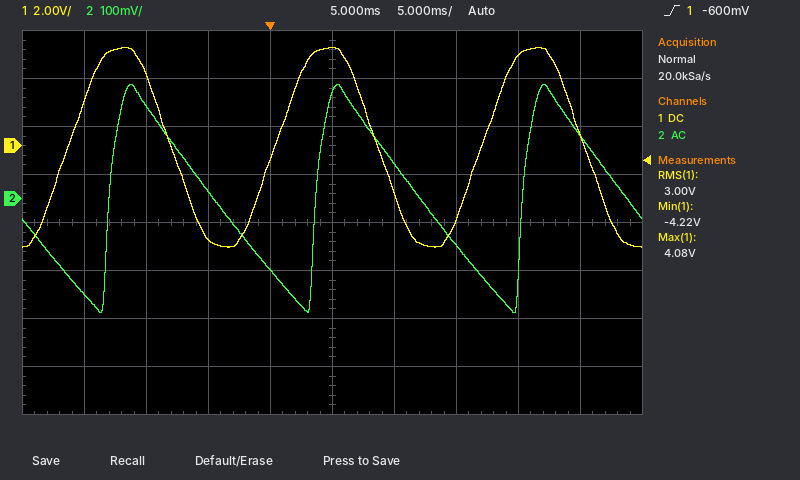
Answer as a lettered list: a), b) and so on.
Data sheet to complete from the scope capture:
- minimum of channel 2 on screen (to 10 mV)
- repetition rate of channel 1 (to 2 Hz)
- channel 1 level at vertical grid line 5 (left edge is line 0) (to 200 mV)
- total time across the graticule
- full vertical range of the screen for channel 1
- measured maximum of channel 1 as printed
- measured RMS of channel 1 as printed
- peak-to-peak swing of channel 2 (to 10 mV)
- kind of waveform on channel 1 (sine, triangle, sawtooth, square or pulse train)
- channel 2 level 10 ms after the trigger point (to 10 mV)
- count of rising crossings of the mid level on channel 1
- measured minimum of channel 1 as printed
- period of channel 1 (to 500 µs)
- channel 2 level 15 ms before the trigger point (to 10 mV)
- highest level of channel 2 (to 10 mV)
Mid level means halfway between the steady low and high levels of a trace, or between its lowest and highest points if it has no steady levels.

a) -240 mV
b) 60 Hz
c) 4.0 V
d) 50 ms
e) 16 V
f) 4.08 V
g) 3.00 V
h) 480 mV
i) sine
j) 70 mV
k) 3
l) -4.22 V
m) 16.5 ms
n) -200 mV
o) 240 mV
